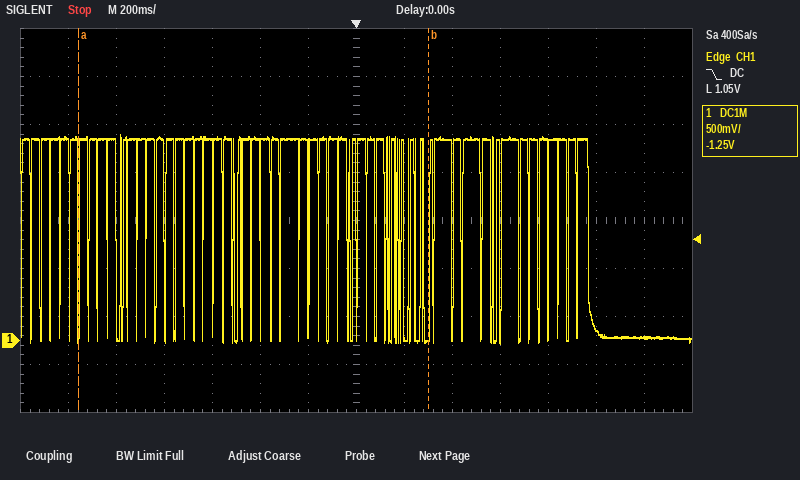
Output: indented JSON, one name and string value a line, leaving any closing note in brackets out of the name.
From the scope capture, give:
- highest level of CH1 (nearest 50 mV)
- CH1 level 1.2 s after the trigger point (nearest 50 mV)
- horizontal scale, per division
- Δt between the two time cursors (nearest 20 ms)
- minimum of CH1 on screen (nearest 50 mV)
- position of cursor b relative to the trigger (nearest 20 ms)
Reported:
{
  "highest level of CH1": "2.15 V",
  "CH1 level 1.2 s after the trigger point": "50 mV",
  "horizontal scale, per division": "200 ms",
  "Δt between the two time cursors": "1.46 s",
  "minimum of CH1 on screen": "-50 mV",
  "position of cursor b relative to the trigger": "+300 ms"
}
